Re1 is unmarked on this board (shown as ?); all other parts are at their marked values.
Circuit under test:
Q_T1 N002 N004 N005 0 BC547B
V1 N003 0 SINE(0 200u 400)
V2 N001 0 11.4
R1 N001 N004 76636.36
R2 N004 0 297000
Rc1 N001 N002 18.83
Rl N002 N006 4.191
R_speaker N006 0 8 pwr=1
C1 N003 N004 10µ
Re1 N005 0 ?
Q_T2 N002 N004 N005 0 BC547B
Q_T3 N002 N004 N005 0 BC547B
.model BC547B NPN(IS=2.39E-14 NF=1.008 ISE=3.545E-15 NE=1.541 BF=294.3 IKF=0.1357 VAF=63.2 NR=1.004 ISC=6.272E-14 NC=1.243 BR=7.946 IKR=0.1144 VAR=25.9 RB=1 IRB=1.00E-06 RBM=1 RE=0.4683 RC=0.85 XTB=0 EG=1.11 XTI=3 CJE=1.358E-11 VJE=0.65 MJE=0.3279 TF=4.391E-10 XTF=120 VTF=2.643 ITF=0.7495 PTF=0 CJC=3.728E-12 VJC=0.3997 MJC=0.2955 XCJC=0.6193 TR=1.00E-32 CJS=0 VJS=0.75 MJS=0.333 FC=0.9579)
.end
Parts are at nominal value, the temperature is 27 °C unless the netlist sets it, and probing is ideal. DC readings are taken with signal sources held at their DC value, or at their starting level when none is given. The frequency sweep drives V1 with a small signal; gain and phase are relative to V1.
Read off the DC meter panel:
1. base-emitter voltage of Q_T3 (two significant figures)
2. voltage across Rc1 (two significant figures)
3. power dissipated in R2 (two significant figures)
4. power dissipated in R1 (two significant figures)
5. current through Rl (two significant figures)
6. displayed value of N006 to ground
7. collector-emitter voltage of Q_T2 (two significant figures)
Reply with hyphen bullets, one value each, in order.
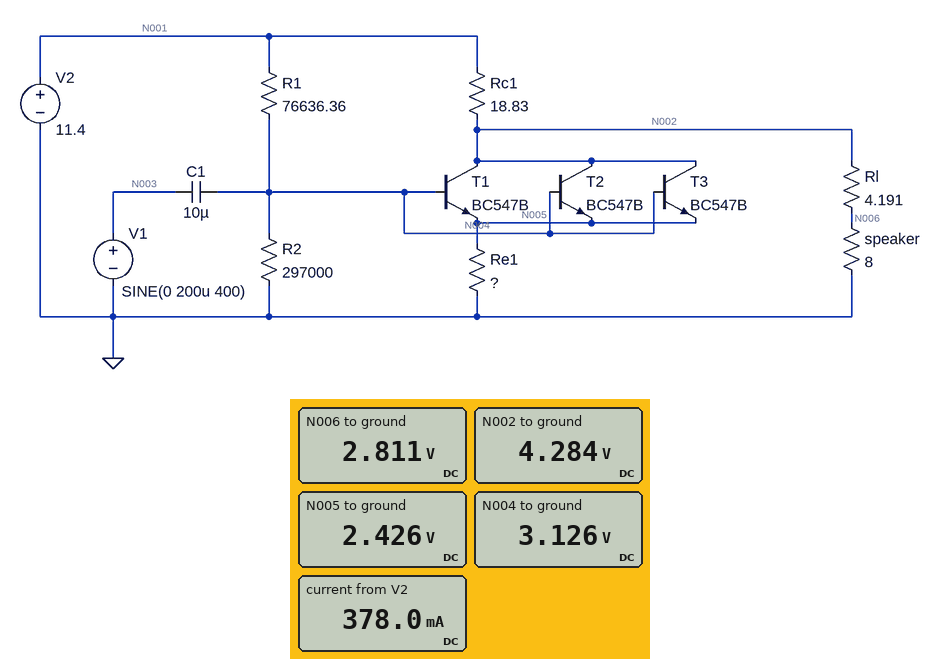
- 700 mV
- 7.1 V
- 33 µW
- 890 µW
- 350 mA
- 2.811 V
- 1.9 V
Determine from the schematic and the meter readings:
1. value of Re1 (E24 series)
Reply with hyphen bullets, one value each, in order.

- 91 Ω
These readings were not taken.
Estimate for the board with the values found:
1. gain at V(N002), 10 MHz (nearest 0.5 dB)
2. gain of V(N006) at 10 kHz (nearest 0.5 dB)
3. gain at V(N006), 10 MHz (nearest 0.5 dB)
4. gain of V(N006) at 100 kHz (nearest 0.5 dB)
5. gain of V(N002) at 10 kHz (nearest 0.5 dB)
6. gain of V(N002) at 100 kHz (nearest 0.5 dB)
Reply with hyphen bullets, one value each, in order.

- -22.0 dB
- -25.5 dB
- -25.5 dB
- -25.5 dB
- -22.0 dB
- -22.0 dB
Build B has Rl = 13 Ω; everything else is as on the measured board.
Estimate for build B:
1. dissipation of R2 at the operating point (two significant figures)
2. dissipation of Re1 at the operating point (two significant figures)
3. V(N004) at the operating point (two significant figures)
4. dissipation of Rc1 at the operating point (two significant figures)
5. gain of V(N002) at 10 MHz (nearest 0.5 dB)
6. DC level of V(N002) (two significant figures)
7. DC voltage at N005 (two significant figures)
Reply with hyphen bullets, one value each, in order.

- 34 µW
- 67 mW
- 3.2 V
- 1.7 W
- -19.5 dB
- 5.7 V
- 2.5 V
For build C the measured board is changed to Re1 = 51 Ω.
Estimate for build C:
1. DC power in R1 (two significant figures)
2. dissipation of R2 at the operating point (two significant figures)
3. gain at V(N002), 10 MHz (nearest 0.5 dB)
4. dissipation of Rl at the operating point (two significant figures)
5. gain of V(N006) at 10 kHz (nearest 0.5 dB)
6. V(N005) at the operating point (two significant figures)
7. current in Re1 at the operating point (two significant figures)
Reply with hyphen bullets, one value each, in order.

- 1.1 mW
- 17 µW
- -17.0 dB
- 510 mW
- -20.5 dB
- 1.6 V
- 31 mA
